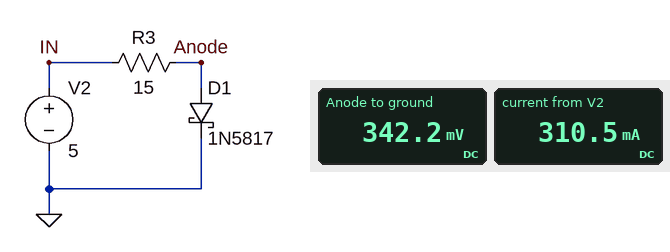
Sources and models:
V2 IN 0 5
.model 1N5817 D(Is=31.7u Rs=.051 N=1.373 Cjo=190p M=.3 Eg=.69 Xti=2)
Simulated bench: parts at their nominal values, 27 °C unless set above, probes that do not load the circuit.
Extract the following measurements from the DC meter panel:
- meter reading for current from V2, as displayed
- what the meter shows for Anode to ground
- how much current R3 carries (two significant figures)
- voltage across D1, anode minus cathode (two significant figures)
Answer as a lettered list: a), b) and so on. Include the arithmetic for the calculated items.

a) 310.5 mA
b) 342.2 mV
c) (5 V - 342.2 mV) / 15 Ω = 310 mA
d) 342.2 mV = 340 mV
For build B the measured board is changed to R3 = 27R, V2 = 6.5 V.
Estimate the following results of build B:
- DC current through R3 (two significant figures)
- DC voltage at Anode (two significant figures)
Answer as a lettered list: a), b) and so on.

a) 230 mA
b) 330 mV
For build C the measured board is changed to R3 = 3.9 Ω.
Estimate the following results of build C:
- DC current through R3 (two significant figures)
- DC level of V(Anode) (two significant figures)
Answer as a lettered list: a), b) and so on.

a) 1.2 A
b) 430 mV
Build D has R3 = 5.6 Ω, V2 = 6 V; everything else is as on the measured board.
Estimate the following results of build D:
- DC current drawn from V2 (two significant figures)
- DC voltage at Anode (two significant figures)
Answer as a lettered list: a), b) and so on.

a) 1.0 A
b) 420 mV
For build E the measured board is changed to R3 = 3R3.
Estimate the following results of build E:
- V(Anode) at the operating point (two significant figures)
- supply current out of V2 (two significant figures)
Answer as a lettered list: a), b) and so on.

a) 450 mV
b) 1.4 A
